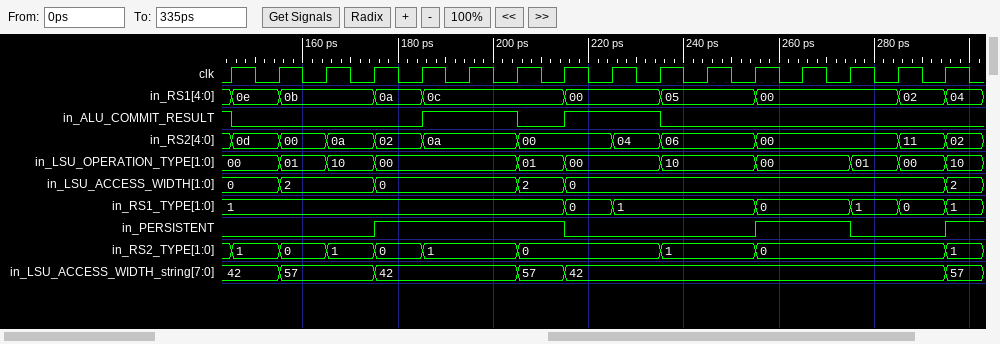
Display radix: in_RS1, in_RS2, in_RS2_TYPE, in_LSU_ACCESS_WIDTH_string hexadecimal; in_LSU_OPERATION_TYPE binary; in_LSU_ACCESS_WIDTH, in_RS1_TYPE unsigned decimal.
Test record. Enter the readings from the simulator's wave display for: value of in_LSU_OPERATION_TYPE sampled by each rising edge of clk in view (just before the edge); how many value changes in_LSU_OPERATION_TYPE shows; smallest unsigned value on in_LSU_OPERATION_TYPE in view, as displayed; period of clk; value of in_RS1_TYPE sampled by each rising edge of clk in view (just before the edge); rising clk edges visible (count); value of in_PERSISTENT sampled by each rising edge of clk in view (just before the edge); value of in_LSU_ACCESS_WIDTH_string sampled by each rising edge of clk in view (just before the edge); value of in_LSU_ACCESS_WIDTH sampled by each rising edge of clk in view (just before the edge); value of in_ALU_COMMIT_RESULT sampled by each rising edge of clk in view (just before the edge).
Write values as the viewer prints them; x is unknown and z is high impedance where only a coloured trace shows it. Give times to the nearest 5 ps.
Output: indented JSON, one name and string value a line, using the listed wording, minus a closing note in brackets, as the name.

{
  "value of in_LSU_OPERATION_TYPE sampled by each rising edge of clk in view": "00, 00, 01, 10, 00, 00, 00, 01, 00, 00, 10, 10, 00, 00, 01, 00",
  "how many value changes in_LSU_OPERATION_TYPE shows": "10",
  "smallest unsigned value on in_LSU_OPERATION_TYPE in view, as displayed": "00",
  "period of clk": "10 ps",
  "value of in_RS1_TYPE sampled by each rising edge of clk in view": "1, 1, 1, 1, 1, 1, 1, 1, 0, 1, 1, 1, 0, 0, 1, 0",
  "rising clk edges visible": "16",
  "value of in_PERSISTENT sampled by each rising edge of clk in view": "0 0 0 0 1 1 1 1 0 0 0 0 1 1 0 0",
  "value of in_LSU_ACCESS_WIDTH_string sampled by each rising edge of clk in view": "42, 42, 57, 57, 42, 42, 42, 57, 42, 42, 42, 42, 42, 42, 42, 42",
  "value of in_LSU_ACCESS_WIDTH sampled by each rising edge of clk in view": "0, 0, 2, 2, 0, 0, 0, 2, 0, 0, 0, 0, 0, 0, 0, 0",
  "value of in_ALU_COMMIT_RESULT sampled by each rising edge of clk in view": "1 0 0 0 0 1 1 0 1 1 0 0 0 0 0 0"
}
